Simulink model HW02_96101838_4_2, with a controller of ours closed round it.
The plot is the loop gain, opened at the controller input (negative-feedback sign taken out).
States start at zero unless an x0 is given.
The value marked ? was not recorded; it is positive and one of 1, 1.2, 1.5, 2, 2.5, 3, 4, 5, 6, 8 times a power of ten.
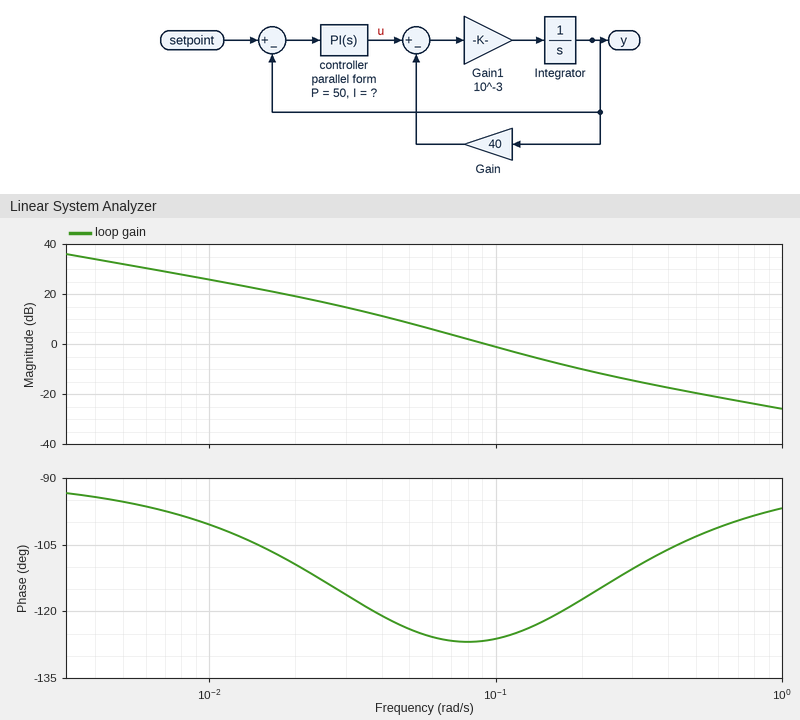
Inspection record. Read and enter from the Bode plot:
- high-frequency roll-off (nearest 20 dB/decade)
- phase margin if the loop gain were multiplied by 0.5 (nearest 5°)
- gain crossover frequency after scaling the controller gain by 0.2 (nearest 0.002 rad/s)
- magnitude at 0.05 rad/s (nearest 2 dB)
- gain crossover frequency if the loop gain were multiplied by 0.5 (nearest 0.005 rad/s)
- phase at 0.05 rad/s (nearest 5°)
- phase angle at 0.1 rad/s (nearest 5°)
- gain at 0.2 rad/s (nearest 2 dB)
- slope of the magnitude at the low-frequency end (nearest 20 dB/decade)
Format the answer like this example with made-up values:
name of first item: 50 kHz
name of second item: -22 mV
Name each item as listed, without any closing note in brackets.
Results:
high-frequency roll-off: -20 dB/decade
phase margin if the loop gain were multiplied by 0.5: 55°
gain crossover frequency after scaling the controller gain by 0.2: 0.032 rad/s
magnitude at 0.05 rad/s: 8 dB
gain crossover frequency if the loop gain were multiplied by 0.5: 0.060 rad/s
phase at 0.05 rad/s: -125°
phase angle at 0.1 rad/s: -125°
gain at 0.2 rad/s: -10 dB
slope of the magnitude at the low-frequency end: -20 dB/decade
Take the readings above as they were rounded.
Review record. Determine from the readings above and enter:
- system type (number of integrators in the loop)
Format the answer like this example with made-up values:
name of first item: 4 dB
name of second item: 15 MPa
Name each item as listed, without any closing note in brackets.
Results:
system type: 1
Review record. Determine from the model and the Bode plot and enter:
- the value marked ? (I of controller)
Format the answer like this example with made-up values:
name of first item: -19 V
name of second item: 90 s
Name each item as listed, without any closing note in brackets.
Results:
the value marked ?: 8
